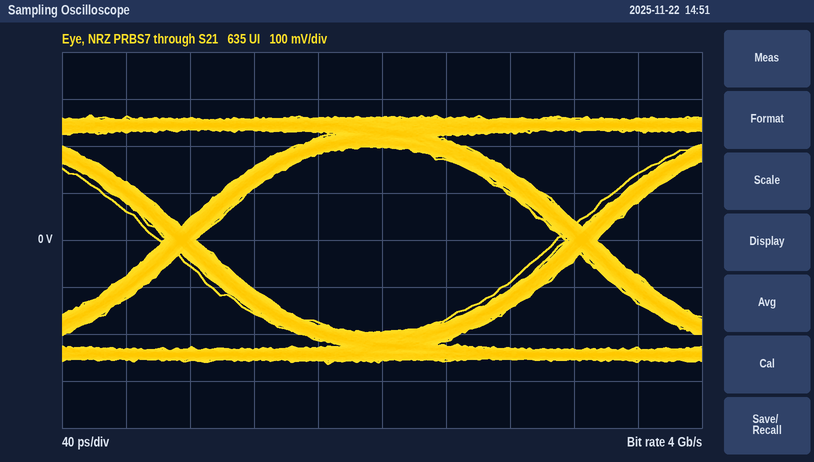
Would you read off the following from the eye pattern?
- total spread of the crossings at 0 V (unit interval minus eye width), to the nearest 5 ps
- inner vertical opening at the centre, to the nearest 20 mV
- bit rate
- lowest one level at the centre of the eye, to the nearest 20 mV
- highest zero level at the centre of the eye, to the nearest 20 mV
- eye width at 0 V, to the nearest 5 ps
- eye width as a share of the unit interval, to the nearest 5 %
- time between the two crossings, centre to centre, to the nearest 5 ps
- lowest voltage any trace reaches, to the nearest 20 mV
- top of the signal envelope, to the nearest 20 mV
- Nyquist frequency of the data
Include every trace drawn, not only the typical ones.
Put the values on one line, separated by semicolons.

25 ps; 400 mV; 4 Gb/s; 200 mV; -200 mV; 225 ps; 90 %; 250 ps; -260 mV; 260 mV; 2 GHz
